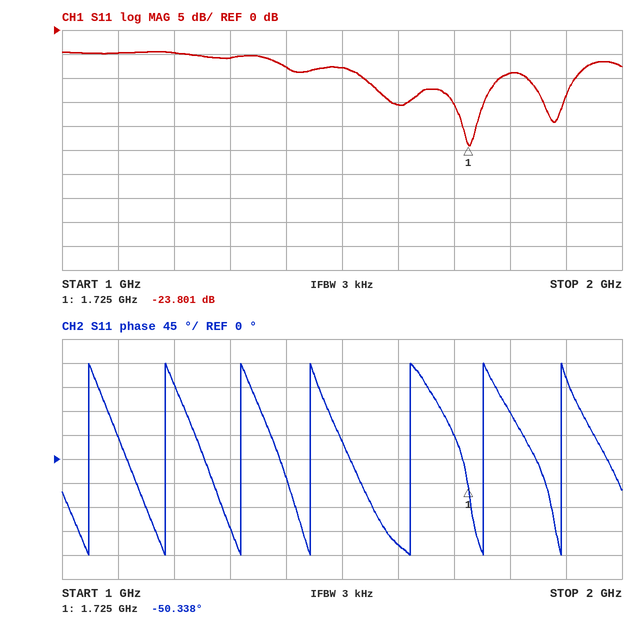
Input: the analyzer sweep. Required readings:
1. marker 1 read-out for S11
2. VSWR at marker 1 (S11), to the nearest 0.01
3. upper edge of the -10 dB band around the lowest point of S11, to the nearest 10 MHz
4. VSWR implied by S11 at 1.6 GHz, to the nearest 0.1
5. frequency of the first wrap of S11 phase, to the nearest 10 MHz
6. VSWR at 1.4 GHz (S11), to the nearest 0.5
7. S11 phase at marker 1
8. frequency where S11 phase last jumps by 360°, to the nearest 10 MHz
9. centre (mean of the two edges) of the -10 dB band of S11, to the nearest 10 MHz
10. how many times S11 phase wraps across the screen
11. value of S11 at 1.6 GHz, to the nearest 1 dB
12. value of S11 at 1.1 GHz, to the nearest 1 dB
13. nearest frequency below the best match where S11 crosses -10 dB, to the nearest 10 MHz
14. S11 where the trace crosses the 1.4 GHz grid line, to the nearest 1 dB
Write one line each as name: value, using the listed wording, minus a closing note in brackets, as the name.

marker 1 read-out for S11: -23.801 dB
VSWR at marker 1 (S11), to the nearest 0.01: 1.14
upper edge of the -10 dB band around the lowest point of S11, to the nearest 10 MHz: 1.78 GHz
VSWR implied by S11 at 1.6 GHz, to the nearest 0.1: 1.4
frequency of the first wrap of S11 phase, to the nearest 10 MHz: 1.05 GHz
VSWR at 1.4 GHz (S11), to the nearest 0.5: 2.5
S11 phase at marker 1: -50.338°
frequency where S11 phase last jumps by 360°, to the nearest 10 MHz: 1.89 GHz
centre (mean of the two edges) of the -10 dB band of S11, to the nearest 10 MHz: 1.66 GHz
how many times S11 phase wraps across the screen: 7
value of S11 at 1.6 GHz, to the nearest 1 dB: -16 dB
value of S11 at 1.1 GHz, to the nearest 1 dB: -5 dB
nearest frequency below the best match where S11 crosses -10 dB, to the nearest 10 MHz: 1.54 GHz
S11 where the trace crosses the 1.4 GHz grid line, to the nearest 1 dB: -8 dB
